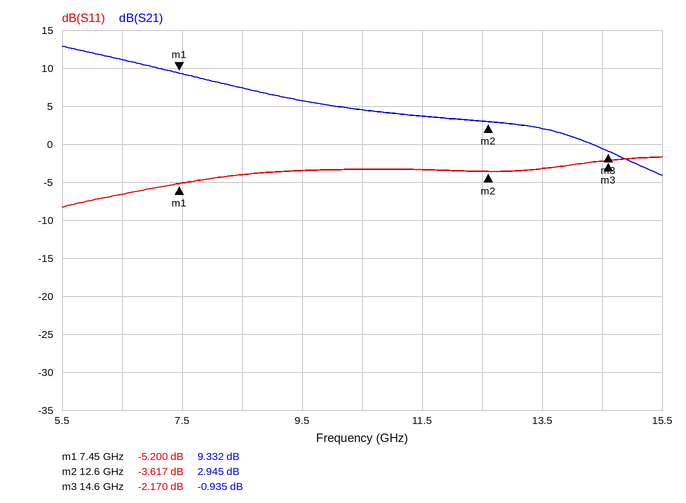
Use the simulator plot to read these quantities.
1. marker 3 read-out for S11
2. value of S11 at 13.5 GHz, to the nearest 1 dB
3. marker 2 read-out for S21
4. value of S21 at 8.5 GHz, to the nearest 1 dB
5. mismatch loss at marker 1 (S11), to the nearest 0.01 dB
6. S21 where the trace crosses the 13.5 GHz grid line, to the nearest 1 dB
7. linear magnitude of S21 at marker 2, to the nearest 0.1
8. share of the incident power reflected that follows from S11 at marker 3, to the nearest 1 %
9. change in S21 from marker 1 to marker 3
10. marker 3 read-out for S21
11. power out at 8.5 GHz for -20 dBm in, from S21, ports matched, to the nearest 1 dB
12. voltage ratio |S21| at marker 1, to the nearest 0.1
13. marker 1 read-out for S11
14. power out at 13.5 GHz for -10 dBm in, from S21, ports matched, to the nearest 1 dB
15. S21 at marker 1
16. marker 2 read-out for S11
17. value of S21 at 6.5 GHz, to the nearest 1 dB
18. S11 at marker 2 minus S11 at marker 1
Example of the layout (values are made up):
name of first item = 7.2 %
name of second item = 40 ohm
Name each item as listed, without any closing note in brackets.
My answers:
marker 3 read-out for S11 = -2.170 dB
value of S11 at 13.5 GHz, to the nearest 1 dB = -3 dB
marker 2 read-out for S21 = 2.945 dB
value of S21 at 8.5 GHz, to the nearest 1 dB = 7 dB
mismatch loss at marker 1 (S11), to the nearest 0.01 dB = 1.56 dB
S21 where the trace crosses the 13.5 GHz grid line, to the nearest 1 dB = 2 dB
linear magnitude of S21 at marker 2, to the nearest 0.1 = 1.4
share of the incident power reflected that follows from S11 at marker 3, to the nearest 1 % = 61 %
change in S21 from marker 1 to marker 3 = -10.267 dB
marker 3 read-out for S21 = -0.935 dB
power out at 8.5 GHz for -20 dBm in, from S21, ports matched, to the nearest 1 dB = -13 dBm
voltage ratio |S21| at marker 1, to the nearest 0.1 = 2.9
marker 1 read-out for S11 = -5.200 dB
power out at 13.5 GHz for -10 dBm in, from S21, ports matched, to the nearest 1 dB = -8 dBm
S21 at marker 1 = 9.332 dB
marker 2 read-out for S11 = -3.617 dB
value of S21 at 6.5 GHz, to the nearest 1 dB = 11 dB
S11 at marker 2 minus S11 at marker 1 = 1.583 dB
